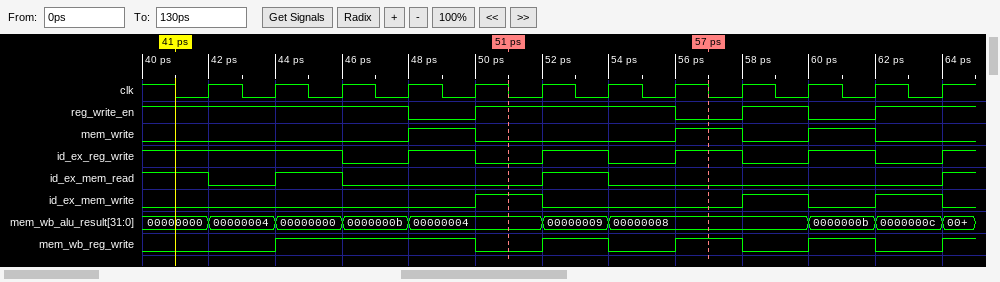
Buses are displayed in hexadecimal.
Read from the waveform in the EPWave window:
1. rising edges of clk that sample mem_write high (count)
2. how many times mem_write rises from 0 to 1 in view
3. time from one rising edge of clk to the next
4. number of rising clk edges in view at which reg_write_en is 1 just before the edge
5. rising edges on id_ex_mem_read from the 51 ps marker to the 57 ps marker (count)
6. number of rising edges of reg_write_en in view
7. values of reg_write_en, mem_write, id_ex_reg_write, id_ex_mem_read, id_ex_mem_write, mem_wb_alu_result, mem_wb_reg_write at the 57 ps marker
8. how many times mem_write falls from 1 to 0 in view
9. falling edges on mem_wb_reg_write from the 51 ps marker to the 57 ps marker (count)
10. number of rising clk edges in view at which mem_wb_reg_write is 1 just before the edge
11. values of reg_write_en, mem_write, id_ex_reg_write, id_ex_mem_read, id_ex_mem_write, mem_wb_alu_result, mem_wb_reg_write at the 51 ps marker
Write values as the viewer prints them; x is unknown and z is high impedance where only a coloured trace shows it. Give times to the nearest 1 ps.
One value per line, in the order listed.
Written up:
3
3
2 ps
9
1
3
reg_write_en=0, mem_write=1, id_ex_reg_write=1, id_ex_mem_read=0, id_ex_mem_write=0, mem_wb_alu_result=00000008, mem_wb_reg_write=1
3
1
6
reg_write_en=1, mem_write=0, id_ex_reg_write=0, id_ex_mem_read=0, id_ex_mem_write=1, mem_wb_alu_result=00000004, mem_wb_reg_write=0
